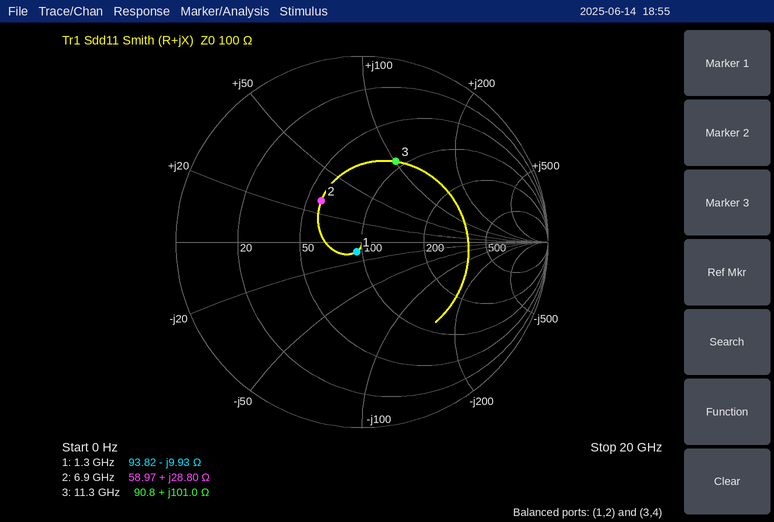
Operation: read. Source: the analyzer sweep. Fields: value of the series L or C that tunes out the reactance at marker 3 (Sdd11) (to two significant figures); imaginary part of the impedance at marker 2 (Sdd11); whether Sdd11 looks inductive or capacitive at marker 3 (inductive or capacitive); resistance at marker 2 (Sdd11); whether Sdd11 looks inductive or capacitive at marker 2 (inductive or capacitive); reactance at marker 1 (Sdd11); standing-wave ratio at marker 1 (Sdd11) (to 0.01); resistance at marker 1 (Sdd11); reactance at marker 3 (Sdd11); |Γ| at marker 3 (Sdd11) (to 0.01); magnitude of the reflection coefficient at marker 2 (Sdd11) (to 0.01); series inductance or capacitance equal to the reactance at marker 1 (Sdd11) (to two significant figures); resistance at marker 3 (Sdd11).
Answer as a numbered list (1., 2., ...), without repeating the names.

1. 140 fF
2. +28.80 Ω
3. inductive
4. 58.97 Ω
5. inductive
6. -9.93 Ω
7. 1.13
8. 93.82 Ω
9. +101.0 Ω
10. 0.47
11. 0.31
12. 12 pF
13. 90.8 Ω
